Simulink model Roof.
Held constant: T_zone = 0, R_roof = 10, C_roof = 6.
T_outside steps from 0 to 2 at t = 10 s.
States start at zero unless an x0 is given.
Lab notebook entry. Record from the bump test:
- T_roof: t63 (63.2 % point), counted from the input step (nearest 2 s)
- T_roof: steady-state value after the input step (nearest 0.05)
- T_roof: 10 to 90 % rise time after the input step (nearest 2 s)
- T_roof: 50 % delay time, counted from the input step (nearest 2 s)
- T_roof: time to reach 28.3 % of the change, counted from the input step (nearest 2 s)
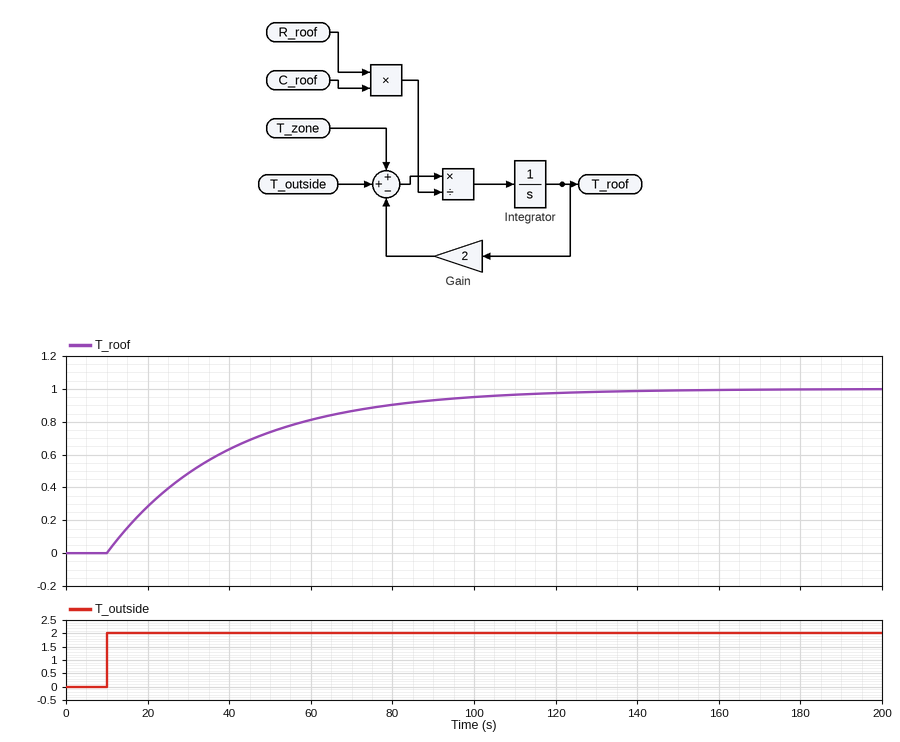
30 s
1.00
66 s
20 s
10 s
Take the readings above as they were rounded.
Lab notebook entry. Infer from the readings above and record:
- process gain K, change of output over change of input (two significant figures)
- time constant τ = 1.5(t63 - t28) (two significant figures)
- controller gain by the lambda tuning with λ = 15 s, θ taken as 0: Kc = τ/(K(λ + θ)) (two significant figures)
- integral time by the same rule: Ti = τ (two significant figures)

0.50
30 s
4.0
30 s
